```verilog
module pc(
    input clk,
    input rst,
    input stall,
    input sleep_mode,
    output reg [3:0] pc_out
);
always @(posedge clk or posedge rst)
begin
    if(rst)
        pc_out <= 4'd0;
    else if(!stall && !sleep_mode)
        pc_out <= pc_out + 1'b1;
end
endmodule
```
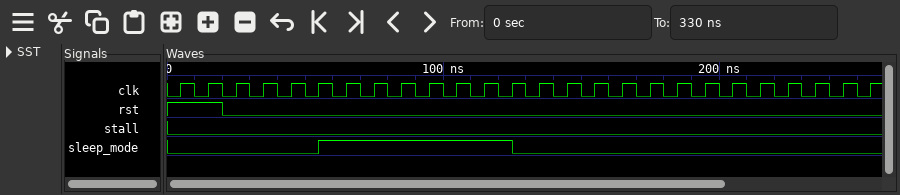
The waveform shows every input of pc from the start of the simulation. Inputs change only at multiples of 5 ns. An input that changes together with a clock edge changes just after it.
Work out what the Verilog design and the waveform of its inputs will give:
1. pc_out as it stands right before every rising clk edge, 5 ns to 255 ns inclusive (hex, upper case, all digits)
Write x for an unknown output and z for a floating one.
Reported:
0, 0, 0, 1, 2, 3, 4, 4, 4, 4, 4, 4, 4, 4, 5, 6, 7, 8, 9, A, B, C, D, E, F, 0
